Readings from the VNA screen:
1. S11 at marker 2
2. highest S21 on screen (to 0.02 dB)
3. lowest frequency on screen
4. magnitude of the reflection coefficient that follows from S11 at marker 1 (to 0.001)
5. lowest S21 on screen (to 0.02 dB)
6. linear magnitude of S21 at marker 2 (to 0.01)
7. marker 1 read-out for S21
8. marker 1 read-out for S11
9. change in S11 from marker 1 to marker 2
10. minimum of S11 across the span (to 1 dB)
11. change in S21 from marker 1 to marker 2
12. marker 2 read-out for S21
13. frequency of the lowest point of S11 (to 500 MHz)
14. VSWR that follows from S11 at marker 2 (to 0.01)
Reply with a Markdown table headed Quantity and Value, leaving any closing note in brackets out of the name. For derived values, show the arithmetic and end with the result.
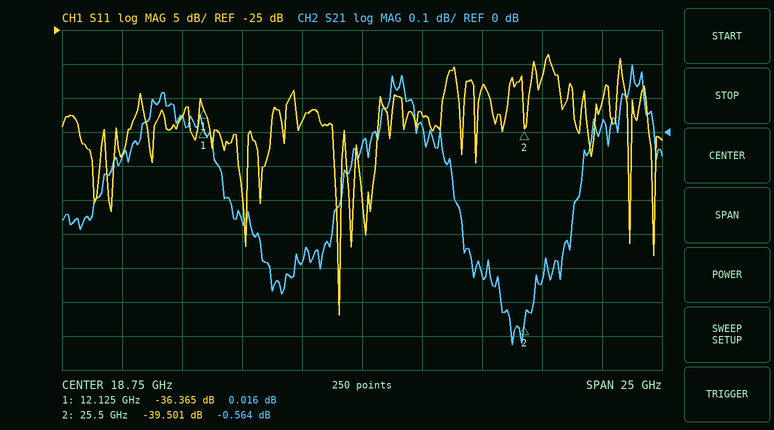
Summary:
| Quantity | Value |
|---|---|
| S11 at marker 2 | -39.501 dB |
| highest S21 on screen | 0.20 dB |
| lowest frequency on screen | 6.25 GHz |
| magnitude of the reflection coefficient that follows from S11 at marker 1 | 10^(-36.365/20) ≈ 0.015 |
| lowest S21 on screen | -0.62 dB |
| linear magnitude of S21 at marker 2 | 10^(-0.564/20) ≈ 0.94 |
| marker 1 read-out for S21 | 0.016 dB |
| marker 1 read-out for S11 | -36.365 dB |
| change in S11 from marker 1 to marker 2 | -39.501 − (-36.365) = -3.136 dB |
| minimum of S11 across the span | -67 dB |
| change in S21 from marker 1 to marker 2 | -0.564 − (0.016) = -0.580 dB |
| marker 2 read-out for S21 | -0.564 dB |
| frequency of the lowest point of S11 | 18.0 GHz |
| VSWR that follows from S11 at marker 2 | (1 + 0.0106)/(1 − 0.0106) ≈ 1.02 |
